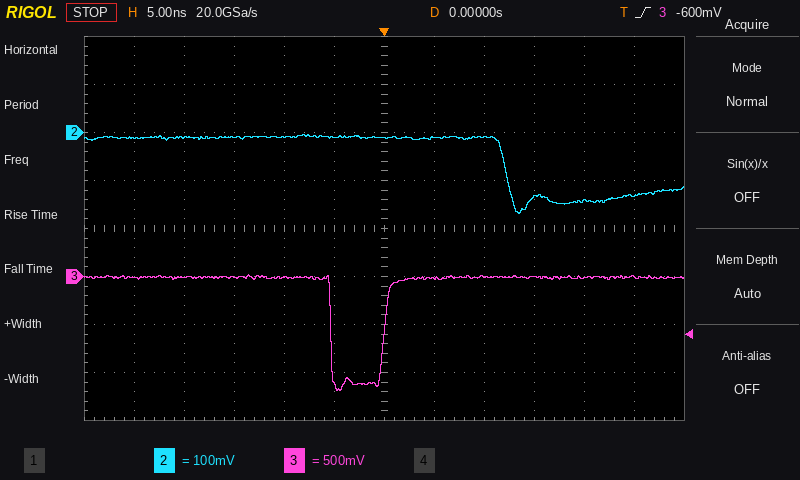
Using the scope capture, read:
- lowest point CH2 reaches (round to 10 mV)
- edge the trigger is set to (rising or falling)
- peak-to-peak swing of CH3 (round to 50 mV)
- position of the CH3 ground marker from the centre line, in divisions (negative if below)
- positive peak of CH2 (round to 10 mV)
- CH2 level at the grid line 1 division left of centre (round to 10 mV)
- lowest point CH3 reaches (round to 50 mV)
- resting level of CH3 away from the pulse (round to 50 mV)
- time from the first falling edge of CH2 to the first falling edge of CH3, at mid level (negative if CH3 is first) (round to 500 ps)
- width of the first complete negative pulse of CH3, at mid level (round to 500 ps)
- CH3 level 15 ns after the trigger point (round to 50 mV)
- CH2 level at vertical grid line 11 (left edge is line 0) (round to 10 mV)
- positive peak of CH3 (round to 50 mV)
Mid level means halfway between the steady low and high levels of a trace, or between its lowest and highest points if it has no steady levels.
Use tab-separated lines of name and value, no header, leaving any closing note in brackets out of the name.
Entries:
lowest point CH2 reaches	-170 mV
edge the trigger is set to	rising
peak-to-peak swing of CH3	1.20 V
position of the CH3 ground marker from the centre line, in divisions	-1.0 div
positive peak of CH2	0 mV
CH2 level at the grid line 1 division left of centre	-10 mV
lowest point CH3 reaches	-1.20 V
resting level of CH3 away from the pulse	0 mV
time from the first falling edge of CH2 to the first falling edge of CH3, at mid level (negative if CH3 is first)	-17.5 ns
width of the first complete negative pulse of CH3, at mid level	5.5 ns
CH3 level 15 ns after the trigger point	0 mV
CH2 level at vertical grid line 11 (left edge is line 0)	-130 mV
positive peak of CH3	0 mV
